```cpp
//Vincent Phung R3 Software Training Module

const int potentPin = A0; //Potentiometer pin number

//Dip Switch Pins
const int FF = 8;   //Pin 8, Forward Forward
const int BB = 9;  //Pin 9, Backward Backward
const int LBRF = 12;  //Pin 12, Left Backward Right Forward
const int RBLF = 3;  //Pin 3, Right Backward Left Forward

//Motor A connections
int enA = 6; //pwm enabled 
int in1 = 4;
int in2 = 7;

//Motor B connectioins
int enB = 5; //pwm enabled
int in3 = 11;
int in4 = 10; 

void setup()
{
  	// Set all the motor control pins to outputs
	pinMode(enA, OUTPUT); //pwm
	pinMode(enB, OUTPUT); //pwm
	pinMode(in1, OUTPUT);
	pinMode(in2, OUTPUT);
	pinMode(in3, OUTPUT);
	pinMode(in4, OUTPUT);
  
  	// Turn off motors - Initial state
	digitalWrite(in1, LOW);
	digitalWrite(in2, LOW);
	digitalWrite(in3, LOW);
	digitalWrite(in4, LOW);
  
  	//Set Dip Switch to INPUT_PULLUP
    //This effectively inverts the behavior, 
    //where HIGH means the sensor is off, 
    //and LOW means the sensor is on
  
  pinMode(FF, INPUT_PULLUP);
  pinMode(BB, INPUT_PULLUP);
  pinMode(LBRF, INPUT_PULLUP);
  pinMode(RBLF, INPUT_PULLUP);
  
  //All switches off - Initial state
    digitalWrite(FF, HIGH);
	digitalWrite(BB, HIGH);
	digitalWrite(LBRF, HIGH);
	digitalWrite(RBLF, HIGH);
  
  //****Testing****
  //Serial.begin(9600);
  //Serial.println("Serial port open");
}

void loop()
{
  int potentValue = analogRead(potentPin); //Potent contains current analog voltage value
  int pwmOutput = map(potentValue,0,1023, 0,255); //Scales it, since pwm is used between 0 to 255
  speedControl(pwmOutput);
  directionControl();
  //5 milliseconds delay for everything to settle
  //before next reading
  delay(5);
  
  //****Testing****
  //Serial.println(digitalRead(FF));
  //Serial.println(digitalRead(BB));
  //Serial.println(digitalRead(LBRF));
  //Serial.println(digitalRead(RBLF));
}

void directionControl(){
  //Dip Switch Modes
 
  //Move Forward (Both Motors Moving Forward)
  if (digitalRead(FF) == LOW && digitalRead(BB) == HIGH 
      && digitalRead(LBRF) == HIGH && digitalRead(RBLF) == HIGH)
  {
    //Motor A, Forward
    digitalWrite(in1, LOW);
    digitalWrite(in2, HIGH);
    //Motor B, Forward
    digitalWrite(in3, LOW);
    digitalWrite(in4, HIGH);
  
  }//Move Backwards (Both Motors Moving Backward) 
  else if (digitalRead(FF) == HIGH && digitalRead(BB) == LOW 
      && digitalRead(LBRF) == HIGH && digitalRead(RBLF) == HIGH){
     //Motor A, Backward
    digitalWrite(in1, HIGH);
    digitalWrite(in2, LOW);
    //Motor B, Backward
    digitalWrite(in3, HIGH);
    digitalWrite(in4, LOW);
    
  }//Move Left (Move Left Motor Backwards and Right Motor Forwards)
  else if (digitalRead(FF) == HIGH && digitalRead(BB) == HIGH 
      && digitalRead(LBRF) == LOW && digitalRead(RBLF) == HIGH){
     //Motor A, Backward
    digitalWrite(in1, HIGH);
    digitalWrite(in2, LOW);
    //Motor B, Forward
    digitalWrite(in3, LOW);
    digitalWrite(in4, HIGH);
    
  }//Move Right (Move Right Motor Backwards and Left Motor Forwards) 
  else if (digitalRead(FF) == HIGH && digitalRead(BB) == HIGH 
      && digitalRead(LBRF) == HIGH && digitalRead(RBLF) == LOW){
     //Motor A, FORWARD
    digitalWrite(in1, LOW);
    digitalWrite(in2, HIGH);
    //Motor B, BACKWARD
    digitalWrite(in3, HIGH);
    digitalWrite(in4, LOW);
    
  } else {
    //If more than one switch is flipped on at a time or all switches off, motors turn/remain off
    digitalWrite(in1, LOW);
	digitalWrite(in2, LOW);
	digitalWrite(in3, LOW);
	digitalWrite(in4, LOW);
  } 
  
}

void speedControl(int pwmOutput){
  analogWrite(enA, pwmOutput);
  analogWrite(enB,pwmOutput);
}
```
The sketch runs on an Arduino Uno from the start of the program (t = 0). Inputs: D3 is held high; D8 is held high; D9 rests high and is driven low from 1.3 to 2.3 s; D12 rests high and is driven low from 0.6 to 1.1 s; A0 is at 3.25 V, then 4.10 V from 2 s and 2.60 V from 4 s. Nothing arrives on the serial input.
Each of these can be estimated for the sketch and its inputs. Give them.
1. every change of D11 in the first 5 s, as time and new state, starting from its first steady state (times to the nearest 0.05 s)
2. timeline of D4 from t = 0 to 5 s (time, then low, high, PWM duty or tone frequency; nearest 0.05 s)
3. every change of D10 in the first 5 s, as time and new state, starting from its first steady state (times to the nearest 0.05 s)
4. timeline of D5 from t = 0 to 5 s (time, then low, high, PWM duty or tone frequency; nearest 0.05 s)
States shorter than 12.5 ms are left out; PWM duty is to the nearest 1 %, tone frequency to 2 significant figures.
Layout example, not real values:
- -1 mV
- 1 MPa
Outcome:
- 0 s low; 1.3 s high; 2.3 s low
- 0 s low; 0.6 s high; 1.1 s low; 1.3 s high; 2.3 s low
- 0 s low; 0.6 s high; 1.1 s low
- 0 s PWM 65 %; 2 s PWM 82 %; 4 s PWM 52 %
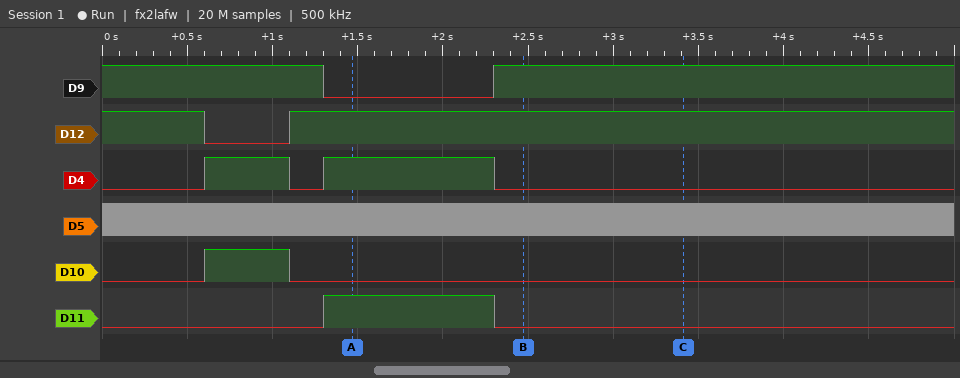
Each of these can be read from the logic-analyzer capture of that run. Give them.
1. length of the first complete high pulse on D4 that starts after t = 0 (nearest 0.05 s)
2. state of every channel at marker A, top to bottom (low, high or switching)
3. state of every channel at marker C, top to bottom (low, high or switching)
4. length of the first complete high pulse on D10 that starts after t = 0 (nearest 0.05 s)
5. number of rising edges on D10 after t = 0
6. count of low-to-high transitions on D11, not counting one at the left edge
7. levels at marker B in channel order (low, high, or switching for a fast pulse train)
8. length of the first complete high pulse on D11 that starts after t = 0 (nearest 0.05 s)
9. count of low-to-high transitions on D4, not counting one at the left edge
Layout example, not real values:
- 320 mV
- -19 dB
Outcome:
- 0.50 s
- D9 low, D12 high, D4 high, D5 switching, D10 low, D11 high
- D9 high, D12 high, D4 low, D5 switching, D10 low, D11 low
- 0.50 s
- 1
- 1
- D9 high, D12 high, D4 low, D5 switching, D10 low, D11 low
- 1.00 s
- 2
